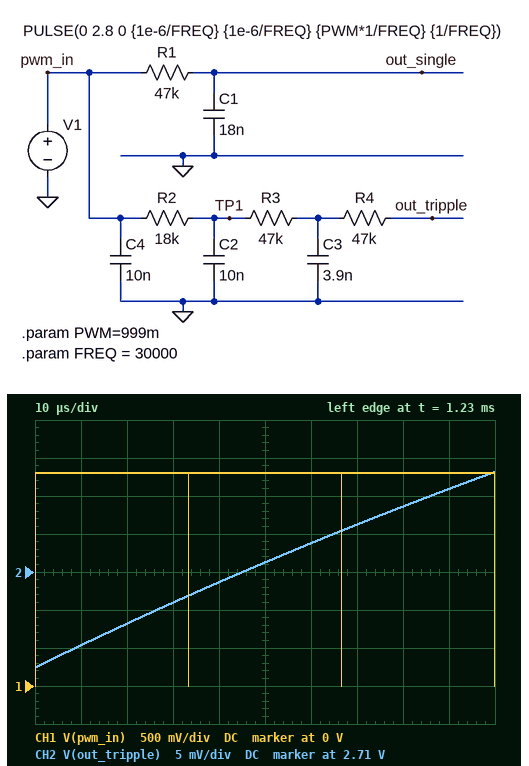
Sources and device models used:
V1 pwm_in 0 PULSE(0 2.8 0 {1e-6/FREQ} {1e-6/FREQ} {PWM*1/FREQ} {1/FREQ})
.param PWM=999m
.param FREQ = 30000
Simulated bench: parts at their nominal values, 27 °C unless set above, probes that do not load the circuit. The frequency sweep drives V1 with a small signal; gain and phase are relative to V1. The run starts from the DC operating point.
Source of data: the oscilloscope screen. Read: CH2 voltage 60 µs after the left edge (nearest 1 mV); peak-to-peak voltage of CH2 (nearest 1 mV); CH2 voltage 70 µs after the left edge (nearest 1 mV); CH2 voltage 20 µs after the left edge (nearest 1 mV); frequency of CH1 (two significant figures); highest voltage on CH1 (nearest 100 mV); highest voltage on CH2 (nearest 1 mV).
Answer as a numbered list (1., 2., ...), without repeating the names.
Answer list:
1. 2.714 V
2. 26 mV
3. 2.716 V
4. 2.703 V
5. 30 kHz
6. 2.8 V
7. 2.723 V
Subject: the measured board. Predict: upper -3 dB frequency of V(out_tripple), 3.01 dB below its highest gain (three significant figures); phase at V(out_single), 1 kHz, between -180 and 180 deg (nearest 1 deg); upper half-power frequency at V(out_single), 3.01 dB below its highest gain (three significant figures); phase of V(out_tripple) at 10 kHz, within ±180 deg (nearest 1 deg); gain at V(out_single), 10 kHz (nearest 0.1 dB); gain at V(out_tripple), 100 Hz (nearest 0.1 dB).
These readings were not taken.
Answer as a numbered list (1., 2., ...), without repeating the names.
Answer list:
1. 441 Hz
2. -79 deg
3. 188 Hz
4. -168 deg
5. -34.5 dB
6. -0.2 dB
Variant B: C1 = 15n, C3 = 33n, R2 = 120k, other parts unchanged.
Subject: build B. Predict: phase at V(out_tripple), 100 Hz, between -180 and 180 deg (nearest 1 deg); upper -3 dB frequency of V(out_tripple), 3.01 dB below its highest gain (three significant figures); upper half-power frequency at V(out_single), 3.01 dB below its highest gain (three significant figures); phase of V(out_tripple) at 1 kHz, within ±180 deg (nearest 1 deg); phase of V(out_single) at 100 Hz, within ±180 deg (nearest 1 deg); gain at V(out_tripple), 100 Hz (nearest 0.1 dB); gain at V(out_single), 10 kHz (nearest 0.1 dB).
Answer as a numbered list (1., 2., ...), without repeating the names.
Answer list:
1. -86 deg
2. 24.7 Hz
3. 226 Hz
4. -150 deg
5. -24 deg
6. -12.5 dB
7. -32.9 dB
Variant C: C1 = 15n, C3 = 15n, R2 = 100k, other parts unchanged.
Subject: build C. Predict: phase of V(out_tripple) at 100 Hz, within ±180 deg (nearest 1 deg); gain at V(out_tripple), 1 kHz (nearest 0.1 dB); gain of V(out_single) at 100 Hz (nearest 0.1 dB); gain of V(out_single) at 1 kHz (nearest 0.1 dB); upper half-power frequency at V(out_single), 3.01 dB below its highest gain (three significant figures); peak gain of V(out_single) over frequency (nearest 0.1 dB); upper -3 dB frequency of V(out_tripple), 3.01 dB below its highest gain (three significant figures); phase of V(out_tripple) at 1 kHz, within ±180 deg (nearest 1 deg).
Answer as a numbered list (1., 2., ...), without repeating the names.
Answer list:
1. -70 deg
2. -30.5 dB
3. -0.8 dB
4. -13.1 dB
5. 226 Hz
6. 0 dB
7. 53.3 Hz
8. -143 deg
